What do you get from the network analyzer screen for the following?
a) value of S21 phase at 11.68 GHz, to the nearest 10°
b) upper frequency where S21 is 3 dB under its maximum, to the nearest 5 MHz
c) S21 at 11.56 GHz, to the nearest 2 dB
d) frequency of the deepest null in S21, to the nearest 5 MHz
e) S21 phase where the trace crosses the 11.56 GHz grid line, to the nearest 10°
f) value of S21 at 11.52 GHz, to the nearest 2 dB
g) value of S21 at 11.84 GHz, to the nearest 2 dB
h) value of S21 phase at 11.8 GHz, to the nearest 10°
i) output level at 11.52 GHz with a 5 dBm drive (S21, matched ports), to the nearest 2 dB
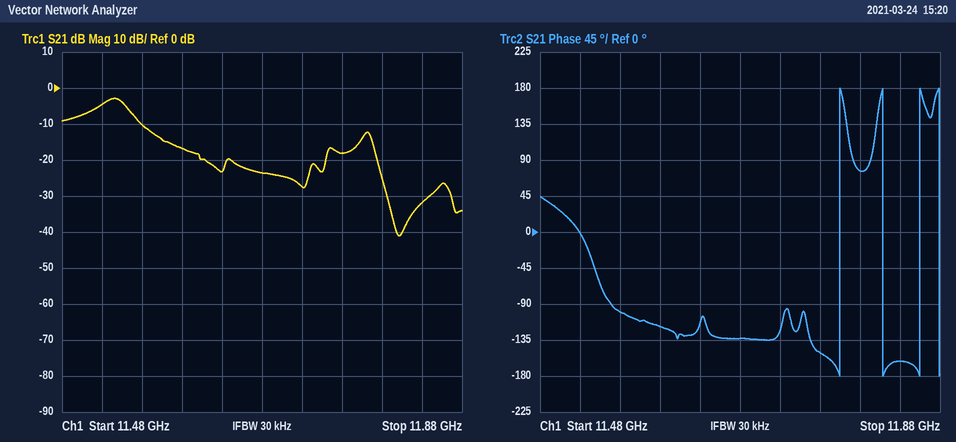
-130°
11.545 GHz
-10 dB
11.815 GHz
-100°
-4 dB
-32 dB
80°
0 dBm
